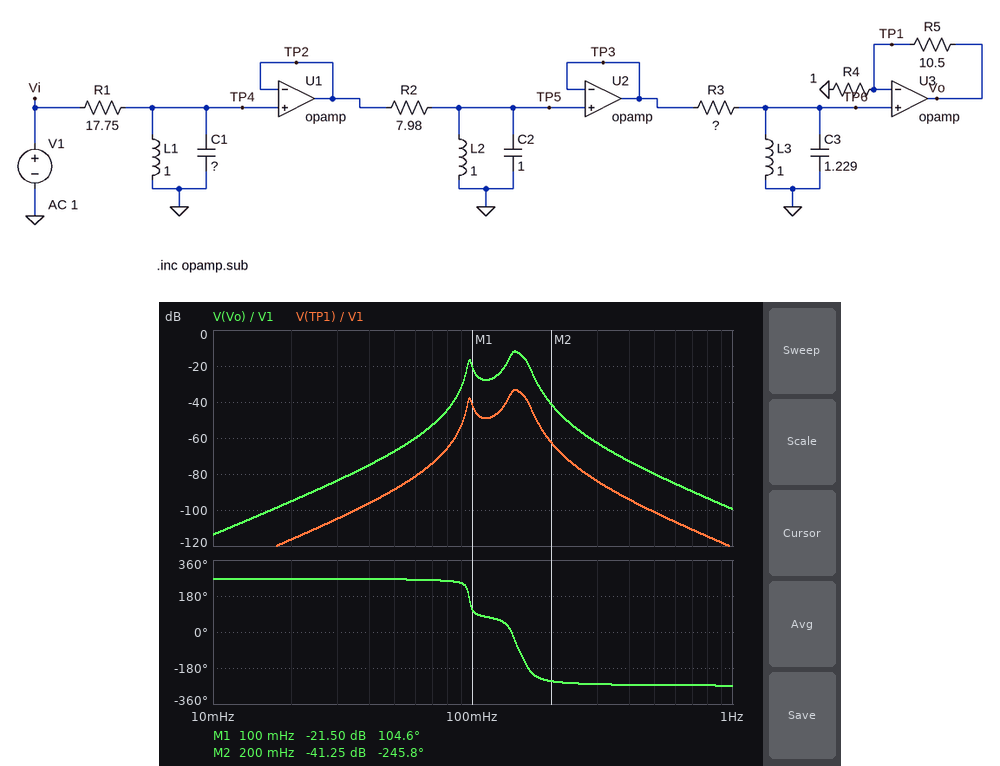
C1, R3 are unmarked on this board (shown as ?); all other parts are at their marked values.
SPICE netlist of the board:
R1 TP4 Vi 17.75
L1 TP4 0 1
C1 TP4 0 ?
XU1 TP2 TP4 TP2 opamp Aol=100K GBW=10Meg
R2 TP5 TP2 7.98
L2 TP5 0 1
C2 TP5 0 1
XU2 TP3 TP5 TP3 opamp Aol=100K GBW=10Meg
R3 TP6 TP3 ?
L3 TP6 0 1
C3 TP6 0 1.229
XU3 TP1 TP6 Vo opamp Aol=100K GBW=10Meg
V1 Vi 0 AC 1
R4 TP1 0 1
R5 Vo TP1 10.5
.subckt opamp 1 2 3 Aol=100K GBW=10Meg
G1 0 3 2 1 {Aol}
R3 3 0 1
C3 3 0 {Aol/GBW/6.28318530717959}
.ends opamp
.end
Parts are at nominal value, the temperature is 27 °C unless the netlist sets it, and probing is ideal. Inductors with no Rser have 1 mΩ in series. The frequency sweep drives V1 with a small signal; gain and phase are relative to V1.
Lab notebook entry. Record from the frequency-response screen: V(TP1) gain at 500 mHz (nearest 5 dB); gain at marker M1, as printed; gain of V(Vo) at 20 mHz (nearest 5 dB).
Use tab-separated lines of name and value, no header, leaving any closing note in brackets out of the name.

V(TP1) gain at 500 mHz	-100 dB
gain at marker M1, as printed	-21.50 dB
gain of V(Vo) at 20 mHz	-95 dB
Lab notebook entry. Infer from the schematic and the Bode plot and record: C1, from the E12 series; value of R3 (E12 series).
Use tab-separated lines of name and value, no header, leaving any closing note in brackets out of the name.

C1, from the E12 series	2.7 F
value of R3	10 Ω
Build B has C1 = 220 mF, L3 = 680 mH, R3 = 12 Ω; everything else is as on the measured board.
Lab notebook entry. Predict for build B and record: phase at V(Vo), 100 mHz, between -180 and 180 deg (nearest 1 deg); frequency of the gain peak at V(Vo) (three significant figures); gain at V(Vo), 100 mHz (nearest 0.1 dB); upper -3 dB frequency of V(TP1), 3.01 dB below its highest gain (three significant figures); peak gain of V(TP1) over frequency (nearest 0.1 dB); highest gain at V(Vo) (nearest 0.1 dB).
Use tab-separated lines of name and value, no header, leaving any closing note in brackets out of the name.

phase at V(Vo), 100 mHz, between -180 and 180 deg	-103 deg
frequency of the gain peak at V(Vo)	173 mHz
gain at V(Vo), 100 mHz	-50.3 dB
upper -3 dB frequency of V(TP1), 3.01 dB below its highest gain	178 mHz
peak gain of V(TP1) over frequency	-26.5 dB
highest gain at V(Vo)	-5.3 dB
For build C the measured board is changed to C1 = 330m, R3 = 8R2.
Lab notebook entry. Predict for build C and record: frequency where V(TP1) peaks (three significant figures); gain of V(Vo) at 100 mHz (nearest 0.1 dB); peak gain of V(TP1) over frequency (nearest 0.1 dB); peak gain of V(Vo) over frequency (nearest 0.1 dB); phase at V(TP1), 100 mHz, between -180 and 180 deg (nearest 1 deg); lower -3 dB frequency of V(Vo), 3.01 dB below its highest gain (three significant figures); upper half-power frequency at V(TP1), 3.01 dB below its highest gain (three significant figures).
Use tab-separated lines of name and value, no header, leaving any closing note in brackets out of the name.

frequency where V(TP1) peaks	153 mHz
gain of V(Vo) at 100 mHz	-41.0 dB
peak gain of V(TP1) over frequency	-27.4 dB
peak gain of V(Vo) over frequency	-6.2 dB
phase at V(TP1), 100 mHz, between -180 and 180 deg	-109 deg
lower -3 dB frequency of V(Vo), 3.01 dB below its highest gain	141 mHz
upper half-power frequency at V(TP1), 3.01 dB below its highest gain	164 mHz
